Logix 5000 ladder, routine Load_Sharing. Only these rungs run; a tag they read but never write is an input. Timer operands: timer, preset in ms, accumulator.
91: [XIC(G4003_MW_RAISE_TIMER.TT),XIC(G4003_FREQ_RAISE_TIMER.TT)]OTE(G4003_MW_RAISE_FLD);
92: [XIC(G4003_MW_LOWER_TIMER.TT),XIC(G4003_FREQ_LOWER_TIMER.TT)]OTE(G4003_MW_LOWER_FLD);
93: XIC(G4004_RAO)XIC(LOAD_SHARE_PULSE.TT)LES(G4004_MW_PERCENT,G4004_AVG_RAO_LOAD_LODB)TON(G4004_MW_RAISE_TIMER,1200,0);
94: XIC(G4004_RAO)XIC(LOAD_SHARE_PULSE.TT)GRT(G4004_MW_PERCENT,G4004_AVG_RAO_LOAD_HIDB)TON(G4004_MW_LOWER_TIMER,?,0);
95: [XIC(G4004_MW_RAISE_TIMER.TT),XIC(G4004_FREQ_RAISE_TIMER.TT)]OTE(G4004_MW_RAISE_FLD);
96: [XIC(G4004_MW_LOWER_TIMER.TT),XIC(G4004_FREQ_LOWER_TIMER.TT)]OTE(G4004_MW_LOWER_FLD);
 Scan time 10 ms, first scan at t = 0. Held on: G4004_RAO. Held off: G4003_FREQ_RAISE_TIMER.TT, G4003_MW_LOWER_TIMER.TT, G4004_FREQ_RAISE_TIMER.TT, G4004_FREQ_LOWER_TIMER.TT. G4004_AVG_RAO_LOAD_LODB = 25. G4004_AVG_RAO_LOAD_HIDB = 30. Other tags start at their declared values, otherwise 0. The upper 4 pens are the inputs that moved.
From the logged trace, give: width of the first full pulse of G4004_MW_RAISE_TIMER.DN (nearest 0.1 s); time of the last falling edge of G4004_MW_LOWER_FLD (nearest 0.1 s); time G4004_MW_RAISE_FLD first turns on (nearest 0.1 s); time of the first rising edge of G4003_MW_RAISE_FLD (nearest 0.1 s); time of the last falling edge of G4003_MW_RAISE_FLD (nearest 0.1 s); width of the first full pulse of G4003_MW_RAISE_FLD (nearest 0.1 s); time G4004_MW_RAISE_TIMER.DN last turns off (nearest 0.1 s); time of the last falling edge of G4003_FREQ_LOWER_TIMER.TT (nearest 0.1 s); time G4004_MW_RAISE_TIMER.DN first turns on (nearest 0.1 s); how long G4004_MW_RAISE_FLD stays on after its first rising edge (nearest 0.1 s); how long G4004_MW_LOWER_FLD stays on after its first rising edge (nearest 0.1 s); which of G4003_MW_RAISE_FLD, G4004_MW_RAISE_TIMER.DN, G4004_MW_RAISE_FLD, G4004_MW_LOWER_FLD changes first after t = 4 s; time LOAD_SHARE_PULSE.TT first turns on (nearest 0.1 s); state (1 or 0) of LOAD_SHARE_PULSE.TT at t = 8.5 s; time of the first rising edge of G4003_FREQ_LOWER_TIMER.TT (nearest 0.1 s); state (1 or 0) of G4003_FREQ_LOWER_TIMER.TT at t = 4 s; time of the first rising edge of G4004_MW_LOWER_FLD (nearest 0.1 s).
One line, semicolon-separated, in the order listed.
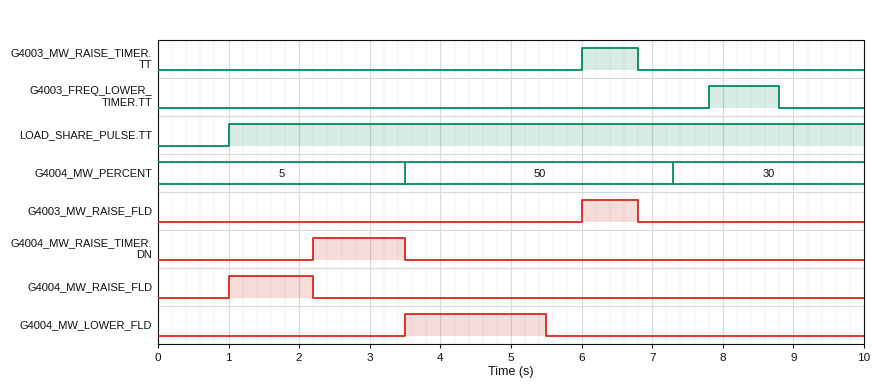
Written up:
1.3 s; 5.5 s; 1.0 s; 6.0 s; 6.8 s; 0.8 s; 3.5 s; 8.8 s; 2.2 s; 1.2 s; 2.0 s; G4004_MW_LOWER_FLD; 1.0 s; 1; 7.8 s; 0; 3.5 s
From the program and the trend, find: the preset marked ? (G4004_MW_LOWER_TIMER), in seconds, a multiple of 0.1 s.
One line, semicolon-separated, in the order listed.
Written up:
2.0 s
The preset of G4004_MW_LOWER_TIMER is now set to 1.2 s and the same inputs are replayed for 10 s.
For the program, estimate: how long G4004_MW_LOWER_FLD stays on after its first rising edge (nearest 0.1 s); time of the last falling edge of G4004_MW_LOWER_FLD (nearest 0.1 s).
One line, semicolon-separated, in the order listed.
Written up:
1.2 s; 4.7 s
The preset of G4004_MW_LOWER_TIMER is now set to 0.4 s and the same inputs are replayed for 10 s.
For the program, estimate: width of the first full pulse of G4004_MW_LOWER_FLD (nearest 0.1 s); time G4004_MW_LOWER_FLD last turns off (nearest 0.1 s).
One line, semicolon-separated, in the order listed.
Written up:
0.4 s; 3.9 s
